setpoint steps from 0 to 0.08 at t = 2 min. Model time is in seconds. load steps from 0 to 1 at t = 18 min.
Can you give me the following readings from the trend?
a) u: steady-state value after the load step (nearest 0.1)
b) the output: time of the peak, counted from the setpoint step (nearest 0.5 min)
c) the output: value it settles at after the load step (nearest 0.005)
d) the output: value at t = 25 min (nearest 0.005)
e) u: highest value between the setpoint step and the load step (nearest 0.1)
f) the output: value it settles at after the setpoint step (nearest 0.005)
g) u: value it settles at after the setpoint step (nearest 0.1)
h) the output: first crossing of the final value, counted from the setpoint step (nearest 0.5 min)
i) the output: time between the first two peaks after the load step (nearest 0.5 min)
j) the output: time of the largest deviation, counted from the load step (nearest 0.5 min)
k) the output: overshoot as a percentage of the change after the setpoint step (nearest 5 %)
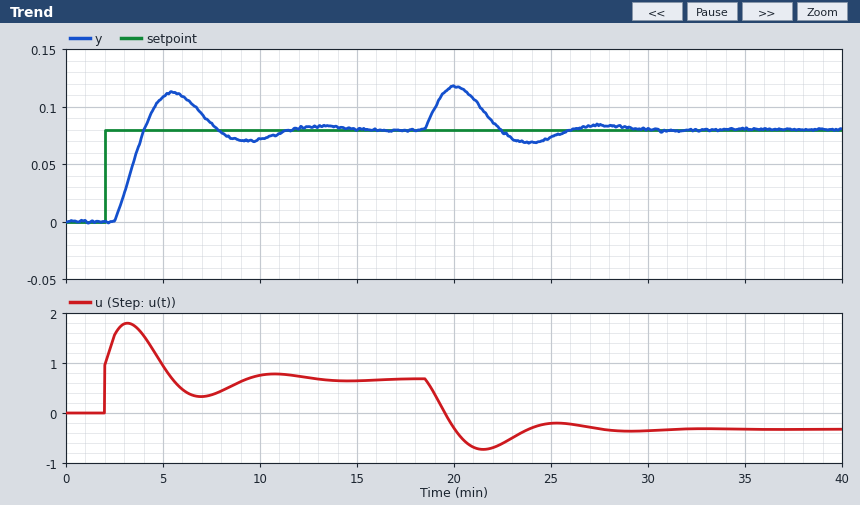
-0.3
3.5 min
0.080
0.075
1.8
0.080
0.7
2.0 min
7.5 min
2.0 min
40 %
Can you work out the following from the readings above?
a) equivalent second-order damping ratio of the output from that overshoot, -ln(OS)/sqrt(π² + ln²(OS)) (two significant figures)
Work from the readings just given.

0.28
